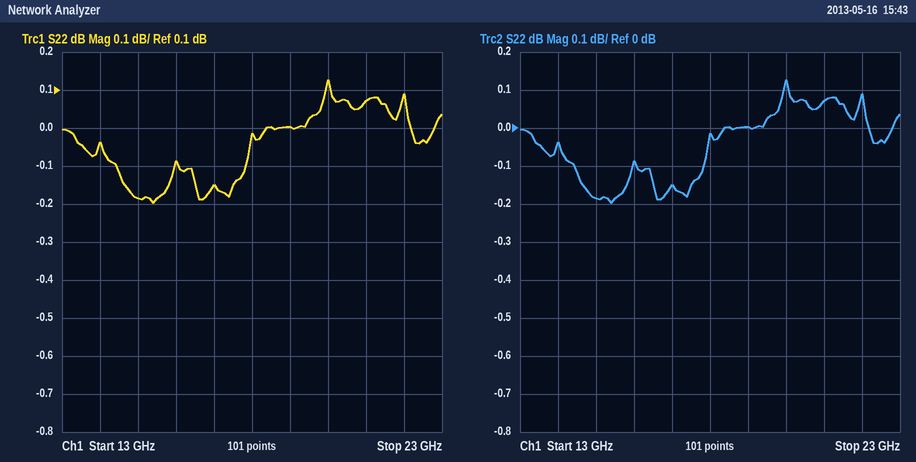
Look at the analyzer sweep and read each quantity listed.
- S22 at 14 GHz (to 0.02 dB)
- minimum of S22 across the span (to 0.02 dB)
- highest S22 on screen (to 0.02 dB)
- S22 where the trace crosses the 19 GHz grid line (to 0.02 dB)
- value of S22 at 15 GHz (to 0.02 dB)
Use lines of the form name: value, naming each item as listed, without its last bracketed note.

S22 at 14 GHz: -0.04 dB
minimum of S22 across the span: -0.20 dB
highest S22 on screen: 0.12 dB
S22 where the trace crosses the 19 GHz grid line: 0.00 dB
value of S22 at 15 GHz: -0.18 dB
